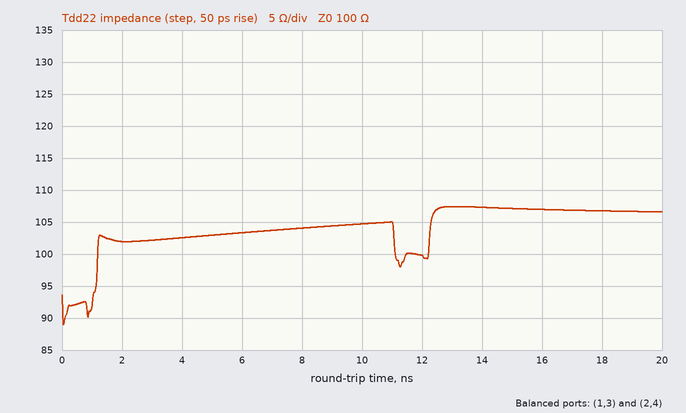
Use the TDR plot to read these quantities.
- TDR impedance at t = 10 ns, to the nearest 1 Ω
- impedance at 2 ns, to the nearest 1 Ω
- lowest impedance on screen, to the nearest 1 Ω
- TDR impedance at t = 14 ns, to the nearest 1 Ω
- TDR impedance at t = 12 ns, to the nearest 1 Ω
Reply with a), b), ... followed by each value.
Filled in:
a) 105 Ω
b) 102 Ω
c) 89 Ω
d) 107 Ω
e) 100 Ω
